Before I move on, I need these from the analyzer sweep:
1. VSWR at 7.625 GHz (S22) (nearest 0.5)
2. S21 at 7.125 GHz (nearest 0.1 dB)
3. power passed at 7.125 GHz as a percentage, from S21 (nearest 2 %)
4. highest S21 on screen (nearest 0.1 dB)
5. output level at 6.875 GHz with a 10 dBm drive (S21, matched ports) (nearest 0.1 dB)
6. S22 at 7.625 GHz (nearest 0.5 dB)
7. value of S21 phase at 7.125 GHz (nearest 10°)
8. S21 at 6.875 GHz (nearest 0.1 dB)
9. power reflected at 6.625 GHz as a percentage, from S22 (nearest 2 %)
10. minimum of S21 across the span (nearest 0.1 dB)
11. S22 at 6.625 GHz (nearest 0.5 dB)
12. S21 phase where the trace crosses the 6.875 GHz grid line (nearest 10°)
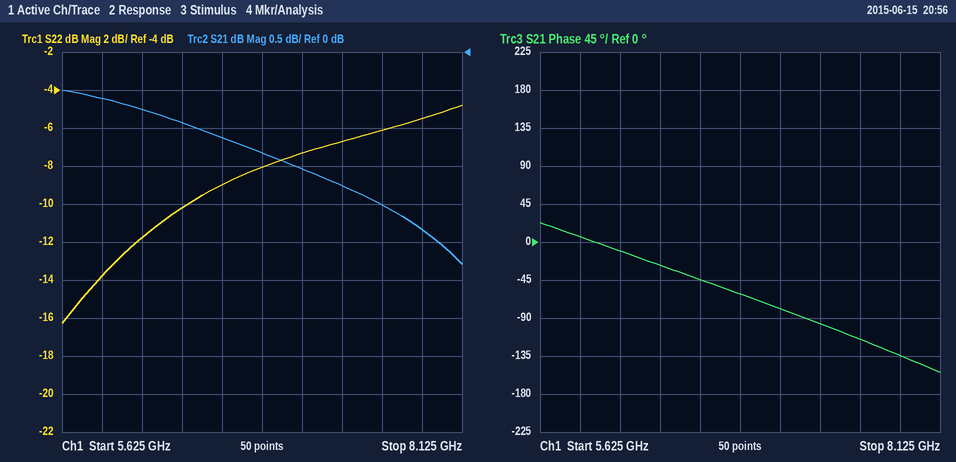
3.0
-1.5 dB
70 %
-0.5 dB
8.7 dBm
-6.0 dB
-80°
-1.3 dB
12 %
-2.8 dB
-9.0 dB
-60°
